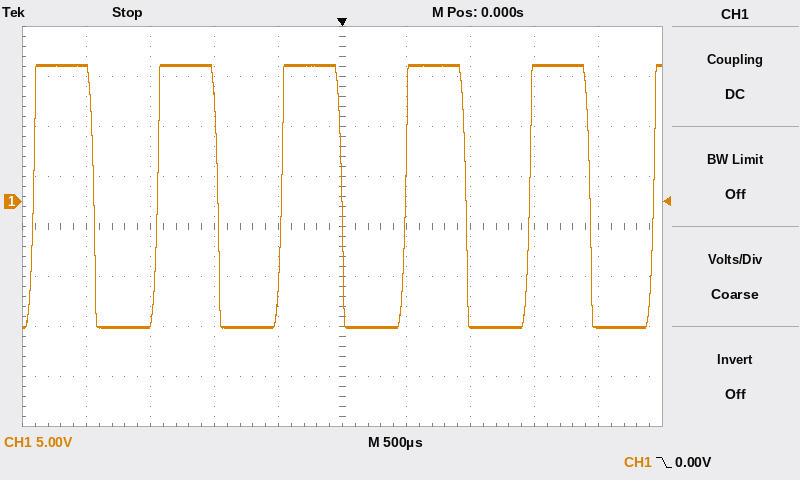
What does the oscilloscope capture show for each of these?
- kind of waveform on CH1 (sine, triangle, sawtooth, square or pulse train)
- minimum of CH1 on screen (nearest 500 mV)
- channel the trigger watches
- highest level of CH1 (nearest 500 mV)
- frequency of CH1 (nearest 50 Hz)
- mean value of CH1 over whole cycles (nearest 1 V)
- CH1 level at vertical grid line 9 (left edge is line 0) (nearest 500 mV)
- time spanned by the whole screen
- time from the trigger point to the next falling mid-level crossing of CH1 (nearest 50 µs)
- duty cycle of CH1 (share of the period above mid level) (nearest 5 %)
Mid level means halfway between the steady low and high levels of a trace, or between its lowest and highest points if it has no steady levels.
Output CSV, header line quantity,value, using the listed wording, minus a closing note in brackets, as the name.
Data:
quantity,value
kind of waveform on CH1,square
minimum of CH1 on screen,-12.5 V
channel the trigger watches,CH1
highest level of CH1,13.5 V
frequency of CH1,1.05 kHz
mean value of CH1 over whole cycles,0 V
CH1 level at vertical grid line 9 (left edge is line 0),-12.5 V
time spanned by the whole screen,5 ms
time from the trigger point to the next falling mid-level crossing of CH1,950 µs
duty cycle of CH1 (share of the period above mid level),50 %
